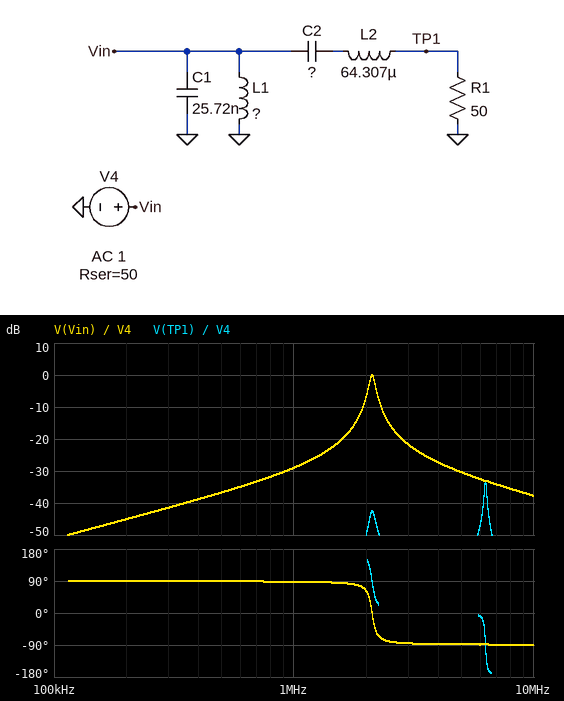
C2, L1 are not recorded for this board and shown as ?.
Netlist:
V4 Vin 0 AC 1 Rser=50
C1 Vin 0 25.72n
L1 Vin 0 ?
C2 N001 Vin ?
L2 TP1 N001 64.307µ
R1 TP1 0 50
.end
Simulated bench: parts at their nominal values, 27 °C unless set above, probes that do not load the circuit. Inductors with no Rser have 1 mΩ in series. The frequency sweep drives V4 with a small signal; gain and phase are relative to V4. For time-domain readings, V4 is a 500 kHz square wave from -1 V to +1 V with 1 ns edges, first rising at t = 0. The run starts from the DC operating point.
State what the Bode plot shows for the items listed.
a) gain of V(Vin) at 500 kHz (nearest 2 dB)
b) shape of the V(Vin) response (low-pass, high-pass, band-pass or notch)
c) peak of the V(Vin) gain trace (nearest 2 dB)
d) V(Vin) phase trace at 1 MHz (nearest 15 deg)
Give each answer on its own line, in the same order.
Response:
-36 dB
band-pass
0 dB
90 deg
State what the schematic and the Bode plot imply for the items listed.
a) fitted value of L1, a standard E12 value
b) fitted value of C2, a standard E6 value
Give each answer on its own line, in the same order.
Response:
220 nH
10 pF
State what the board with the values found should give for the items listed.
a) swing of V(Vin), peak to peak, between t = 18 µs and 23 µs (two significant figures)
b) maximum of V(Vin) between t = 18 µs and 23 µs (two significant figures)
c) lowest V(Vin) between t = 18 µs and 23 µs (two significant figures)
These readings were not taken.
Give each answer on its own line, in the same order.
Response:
140 mV
70 mV
-70 mV
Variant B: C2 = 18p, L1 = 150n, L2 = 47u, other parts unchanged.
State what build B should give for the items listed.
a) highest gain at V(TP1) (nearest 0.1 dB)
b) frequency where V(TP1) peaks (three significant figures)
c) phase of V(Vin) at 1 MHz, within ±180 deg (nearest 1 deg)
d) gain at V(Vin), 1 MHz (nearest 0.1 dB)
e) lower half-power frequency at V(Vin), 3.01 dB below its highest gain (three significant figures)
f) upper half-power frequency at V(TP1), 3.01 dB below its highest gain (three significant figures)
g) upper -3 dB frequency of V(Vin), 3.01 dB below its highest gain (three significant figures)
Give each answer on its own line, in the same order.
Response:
-30.8 dB
5.47 MHz
89 deg
-33.1 dB
2.50 MHz
5.56 MHz
2.62 MHz
